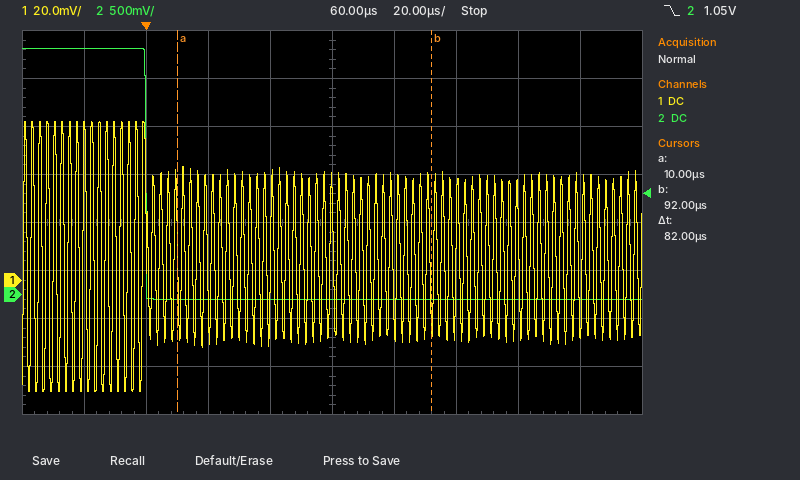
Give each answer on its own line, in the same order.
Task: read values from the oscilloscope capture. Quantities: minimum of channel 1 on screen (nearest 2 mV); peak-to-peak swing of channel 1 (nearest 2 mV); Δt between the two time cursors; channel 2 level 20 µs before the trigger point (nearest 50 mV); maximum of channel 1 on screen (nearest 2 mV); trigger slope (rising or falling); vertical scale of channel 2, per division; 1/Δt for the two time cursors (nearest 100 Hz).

-46 mV
112 mV
82 µs
2.55 V
66 mV
falling
500 mV
12.2 kHz
